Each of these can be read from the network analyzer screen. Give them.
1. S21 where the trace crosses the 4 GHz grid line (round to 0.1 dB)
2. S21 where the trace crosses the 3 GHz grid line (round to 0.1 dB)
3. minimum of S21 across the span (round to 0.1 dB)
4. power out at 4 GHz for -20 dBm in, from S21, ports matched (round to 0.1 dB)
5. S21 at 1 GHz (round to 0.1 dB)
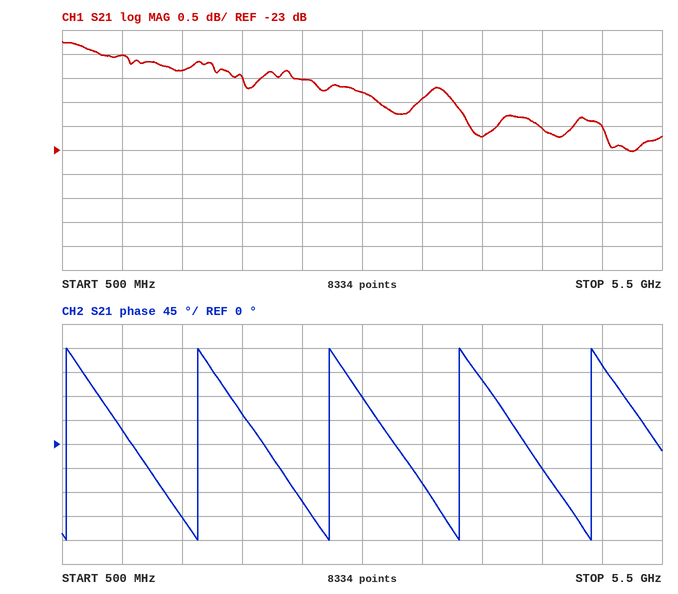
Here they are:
-22.7 dB
-21.8 dB
-23.0 dB
-42.7 dBm
-21.0 dB
